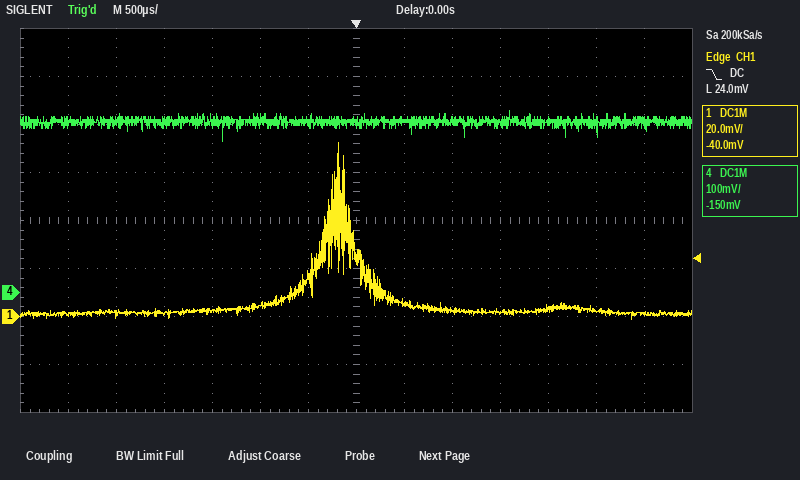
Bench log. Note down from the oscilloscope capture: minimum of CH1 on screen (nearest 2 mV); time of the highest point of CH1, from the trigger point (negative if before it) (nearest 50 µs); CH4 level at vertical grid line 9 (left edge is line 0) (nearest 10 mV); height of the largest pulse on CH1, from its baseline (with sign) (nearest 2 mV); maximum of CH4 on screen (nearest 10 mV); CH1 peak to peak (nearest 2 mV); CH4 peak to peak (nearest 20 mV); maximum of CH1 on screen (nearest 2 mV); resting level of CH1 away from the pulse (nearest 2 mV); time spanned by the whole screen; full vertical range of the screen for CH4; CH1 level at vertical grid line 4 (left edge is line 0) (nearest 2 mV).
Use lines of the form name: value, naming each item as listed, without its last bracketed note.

minimum of CH1 on screen: -2 mV
time of the highest point of CH1, from the trigger point (negative if before it): -200 µs
CH4 level at vertical grid line 9 (left edge is line 0): 360 mV
height of the largest pulse on CH1, from its baseline (with sign): +70 mV
maximum of CH4 on screen: 380 mV
CH1 peak to peak: 74 mV
CH4 peak to peak: 60 mV
maximum of CH1 on screen: 72 mV
resting level of CH1 away from the pulse: 2 mV
time spanned by the whole screen: 7 ms
full vertical range of the screen for CH4: 800 mV
CH1 level at vertical grid line 4 (left edge is line 0): 2 mV
